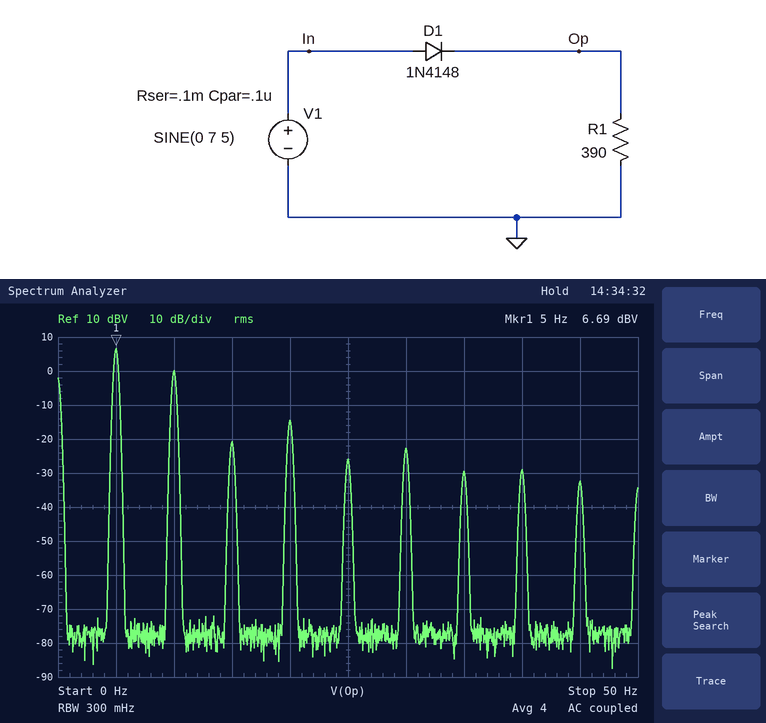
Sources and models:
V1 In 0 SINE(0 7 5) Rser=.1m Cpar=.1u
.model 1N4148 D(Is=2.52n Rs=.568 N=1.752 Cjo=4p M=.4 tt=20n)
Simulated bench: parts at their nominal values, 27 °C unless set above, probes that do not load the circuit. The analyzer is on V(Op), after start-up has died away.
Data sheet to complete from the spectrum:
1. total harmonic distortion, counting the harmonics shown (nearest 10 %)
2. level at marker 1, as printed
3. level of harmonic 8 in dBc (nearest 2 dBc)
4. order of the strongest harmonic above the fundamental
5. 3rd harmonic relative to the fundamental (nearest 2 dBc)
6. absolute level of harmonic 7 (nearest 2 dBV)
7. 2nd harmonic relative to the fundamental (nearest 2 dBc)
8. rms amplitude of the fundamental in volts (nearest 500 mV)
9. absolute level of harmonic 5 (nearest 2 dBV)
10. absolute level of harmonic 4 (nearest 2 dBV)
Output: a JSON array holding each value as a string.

["50 %", "6.69 dBV", "-36 dBc", "2", "-28 dBc", "-30 dBV", "-6 dBc", "2.0 V", "-26 dBV", "-14 dBV"]
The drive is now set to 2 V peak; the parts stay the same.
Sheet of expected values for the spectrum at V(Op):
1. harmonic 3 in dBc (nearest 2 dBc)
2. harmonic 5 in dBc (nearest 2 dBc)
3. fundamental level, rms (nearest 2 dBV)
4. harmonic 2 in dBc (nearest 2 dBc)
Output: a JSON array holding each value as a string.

["-16 dBc", "-24 dBc", "-8 dBV", "-4 dBc"]
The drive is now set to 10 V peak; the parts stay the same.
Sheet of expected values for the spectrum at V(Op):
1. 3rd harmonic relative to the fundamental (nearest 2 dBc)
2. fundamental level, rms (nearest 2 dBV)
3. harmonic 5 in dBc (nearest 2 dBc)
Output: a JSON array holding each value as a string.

["-30 dBc", "10 dBV", "-36 dBc"]
